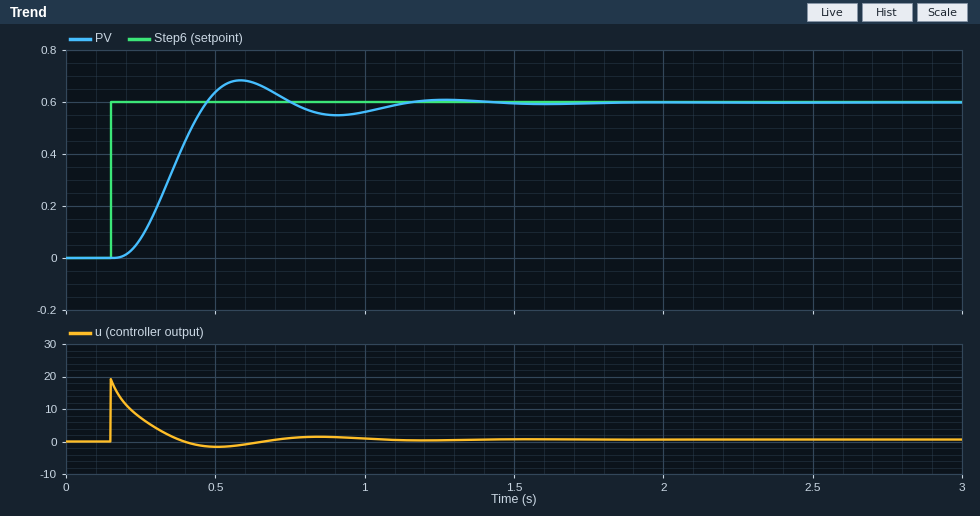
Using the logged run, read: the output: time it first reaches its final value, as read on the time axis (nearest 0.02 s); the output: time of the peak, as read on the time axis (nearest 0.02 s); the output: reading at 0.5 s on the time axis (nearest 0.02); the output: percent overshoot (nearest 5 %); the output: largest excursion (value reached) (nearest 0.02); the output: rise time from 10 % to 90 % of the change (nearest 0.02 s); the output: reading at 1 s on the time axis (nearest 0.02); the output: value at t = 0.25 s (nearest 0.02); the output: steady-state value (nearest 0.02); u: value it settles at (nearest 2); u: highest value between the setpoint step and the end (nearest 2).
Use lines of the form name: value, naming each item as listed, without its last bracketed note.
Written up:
the output: time it first reaches its final value, as read on the time axis: 0.48 s
the output: time of the peak, as read on the time axis: 0.58 s
the output: reading at 0.5 s on the time axis: 0.64
the output: percent overshoot: 15 %
the output: largest excursion (value reached): 0.68
the output: rise time from 10 % to 90 % of the change: 0.20 s
the output: reading at 1 s on the time axis: 0.56
the output: value at t = 0.25 s: 0.08
the output: steady-state value: 0.60
u: value it settles at: 0
u: highest value between the setpoint step and the end: 20
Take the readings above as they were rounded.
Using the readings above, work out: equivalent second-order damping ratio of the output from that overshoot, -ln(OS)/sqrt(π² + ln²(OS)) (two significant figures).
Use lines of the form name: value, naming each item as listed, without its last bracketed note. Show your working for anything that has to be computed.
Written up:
equivalent second-order damping ratio of the output from that overshoot, -ln(OS)/sqrt(π² + ln²(OS)): ln(0.15) = -1.897; 1.897 / sqrt(9.870 + 3.599) = 0.52
